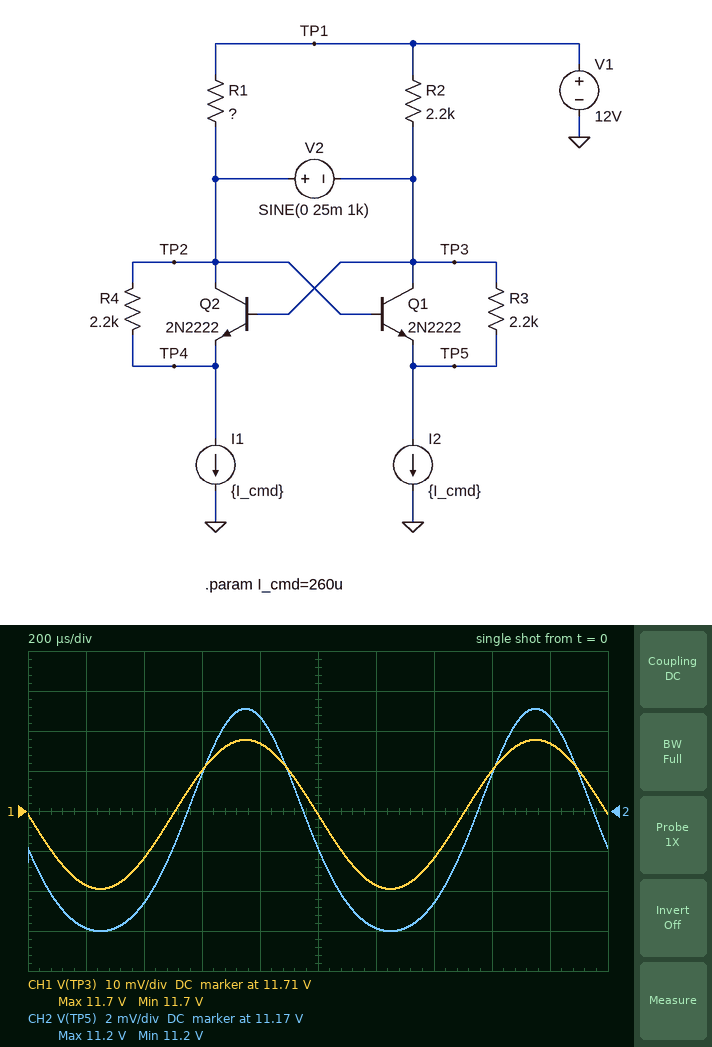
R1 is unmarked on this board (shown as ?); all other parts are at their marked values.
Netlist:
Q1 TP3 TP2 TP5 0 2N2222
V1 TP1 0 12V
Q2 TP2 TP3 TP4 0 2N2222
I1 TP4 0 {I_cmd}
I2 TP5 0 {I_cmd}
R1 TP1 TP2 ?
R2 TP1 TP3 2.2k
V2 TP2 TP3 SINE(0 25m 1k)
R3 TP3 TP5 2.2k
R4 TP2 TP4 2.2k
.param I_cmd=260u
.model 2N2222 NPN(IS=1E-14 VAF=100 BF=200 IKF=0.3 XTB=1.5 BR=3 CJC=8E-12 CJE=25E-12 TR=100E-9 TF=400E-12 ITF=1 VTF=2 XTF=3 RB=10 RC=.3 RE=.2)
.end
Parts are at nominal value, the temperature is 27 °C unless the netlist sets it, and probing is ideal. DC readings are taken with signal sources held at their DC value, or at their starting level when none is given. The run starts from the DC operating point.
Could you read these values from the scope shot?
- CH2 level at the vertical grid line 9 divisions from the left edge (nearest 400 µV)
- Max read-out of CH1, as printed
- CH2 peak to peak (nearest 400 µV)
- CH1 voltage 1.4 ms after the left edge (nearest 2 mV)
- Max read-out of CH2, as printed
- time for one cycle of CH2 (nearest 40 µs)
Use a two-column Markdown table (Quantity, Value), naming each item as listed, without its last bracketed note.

| Quantity | Value |
|---|---|
| CH2 level at the vertical grid line 9 divisions from the left edge | 11.1728 V |
| Max read-out of CH1, as printed | 11.7 V |
| CH2 peak to peak | 11.2 mV |
| CH1 voltage 1.4 ms after the left edge | 11.698 V |
| Max read-out of CH2, as printed | 11.2 V |
| time for one cycle of CH2 | 1.00 ms |
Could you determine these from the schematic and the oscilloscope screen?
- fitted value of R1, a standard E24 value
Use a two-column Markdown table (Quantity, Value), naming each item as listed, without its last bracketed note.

| Quantity | Value |
|---|---|
| fitted value of R1, a standard E24 value | 750 Ω |
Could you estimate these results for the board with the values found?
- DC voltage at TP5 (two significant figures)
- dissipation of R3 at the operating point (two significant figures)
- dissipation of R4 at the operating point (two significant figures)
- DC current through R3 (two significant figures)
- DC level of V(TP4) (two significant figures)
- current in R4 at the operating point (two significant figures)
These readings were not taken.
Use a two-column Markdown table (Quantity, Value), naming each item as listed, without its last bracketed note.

| Quantity | Value |
|---|---|
| DC voltage at TP5 | 11 V |
| dissipation of R3 at the operating point | 130 µW |
| dissipation of R4 at the operating point | 130 µW |
| DC current through R3 | 250 µA |
| DC level of V(TP4) | 11 V |
| current in R4 at the operating point | 250 µA |
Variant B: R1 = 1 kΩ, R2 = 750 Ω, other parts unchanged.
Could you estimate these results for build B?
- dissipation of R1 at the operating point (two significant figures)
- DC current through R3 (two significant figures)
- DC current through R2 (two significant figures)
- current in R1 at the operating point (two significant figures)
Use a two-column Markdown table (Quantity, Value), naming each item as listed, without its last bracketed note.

| Quantity | Value |
|---|---|
| dissipation of R1 at the operating point | 50 µW |
| DC current through R3 | 250 µA |
| DC current through R2 | 300 µA |
| current in R1 at the operating point | 220 µA |
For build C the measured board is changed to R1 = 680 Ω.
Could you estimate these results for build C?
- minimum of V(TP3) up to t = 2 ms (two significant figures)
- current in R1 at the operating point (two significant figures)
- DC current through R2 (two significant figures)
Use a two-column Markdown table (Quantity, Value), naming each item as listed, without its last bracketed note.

| Quantity | Value |
|---|---|
| minimum of V(TP3) up to t = 2 ms | 12 V |
| current in R1 at the operating point | 400 µA |
| DC current through R2 | 120 µA |
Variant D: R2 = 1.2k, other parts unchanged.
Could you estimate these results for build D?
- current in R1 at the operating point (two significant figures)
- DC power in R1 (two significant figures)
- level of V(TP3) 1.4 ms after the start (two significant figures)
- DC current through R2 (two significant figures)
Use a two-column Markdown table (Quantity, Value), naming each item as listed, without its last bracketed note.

| Quantity | Value |
|---|---|
| current in R1 at the operating point | 320 µA |
| DC power in R1 | 77 µW |
| level of V(TP3) 1.4 ms after the start | 12 V |
| DC current through R2 | 200 µA |
